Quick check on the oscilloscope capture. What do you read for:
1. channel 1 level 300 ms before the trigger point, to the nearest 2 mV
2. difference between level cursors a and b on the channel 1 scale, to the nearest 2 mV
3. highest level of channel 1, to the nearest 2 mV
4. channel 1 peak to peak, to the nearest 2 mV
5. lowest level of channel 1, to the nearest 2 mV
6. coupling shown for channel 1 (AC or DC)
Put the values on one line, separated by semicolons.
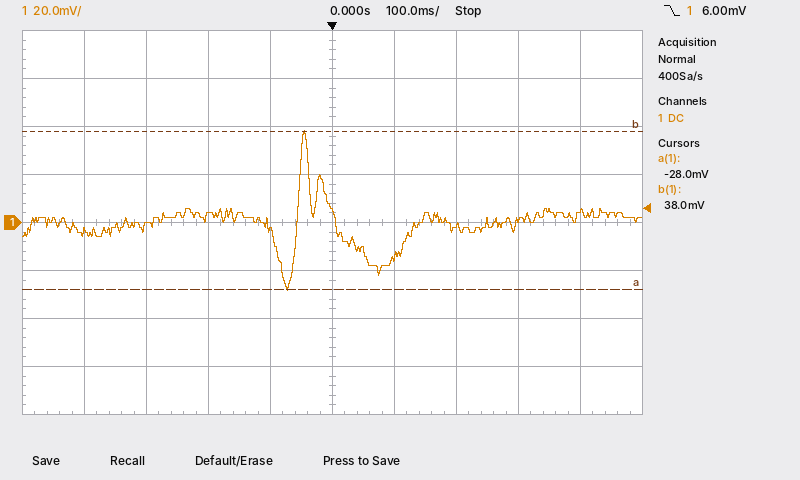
-2 mV; 66 mV; 38 mV; 66 mV; -28 mV; DC
